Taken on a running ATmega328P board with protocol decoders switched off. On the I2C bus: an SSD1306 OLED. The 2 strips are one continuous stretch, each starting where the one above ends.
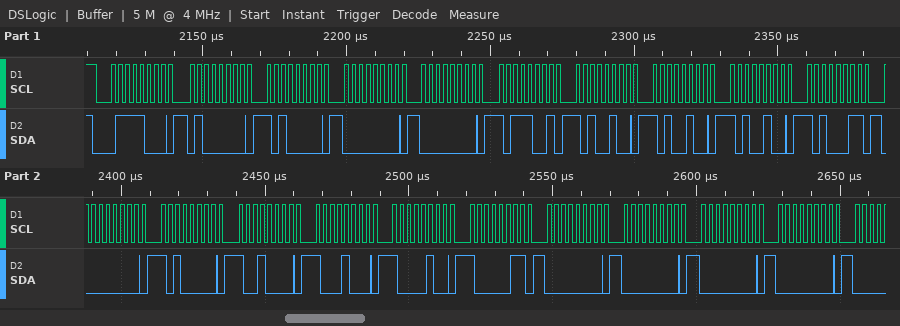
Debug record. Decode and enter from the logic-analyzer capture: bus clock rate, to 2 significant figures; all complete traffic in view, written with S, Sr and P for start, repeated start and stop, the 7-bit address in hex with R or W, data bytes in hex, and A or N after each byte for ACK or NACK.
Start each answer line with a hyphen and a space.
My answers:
- 400 kHz
- S 3CW A 40 A A0 A 00 A 00 A B9 A A4 A A4 A A4 A A3 A 00 A A0 A 90 A 88 A 84 A 83 A 00 A 00 A 00 A 00 A
